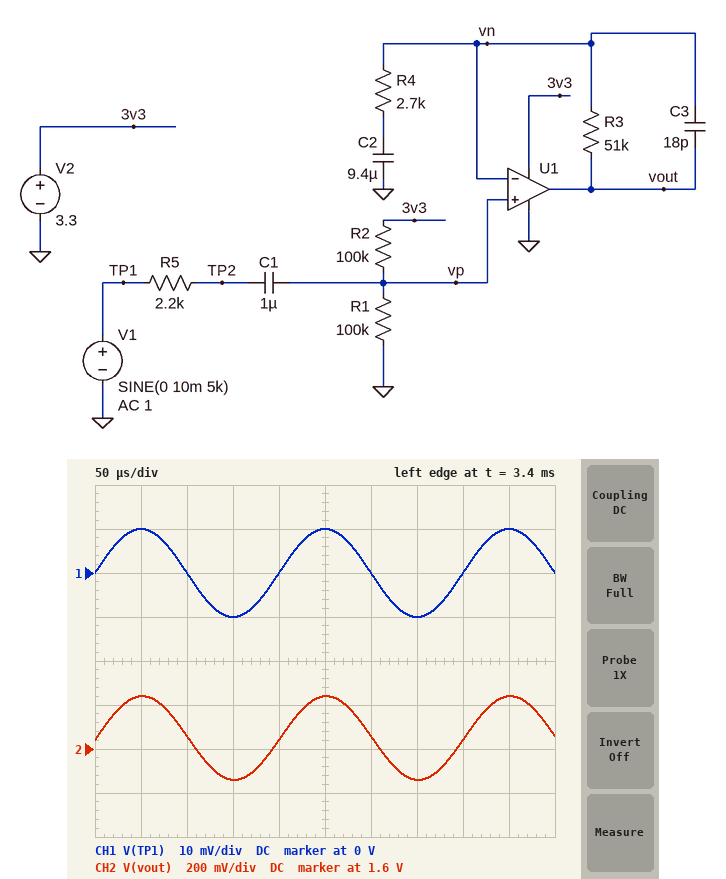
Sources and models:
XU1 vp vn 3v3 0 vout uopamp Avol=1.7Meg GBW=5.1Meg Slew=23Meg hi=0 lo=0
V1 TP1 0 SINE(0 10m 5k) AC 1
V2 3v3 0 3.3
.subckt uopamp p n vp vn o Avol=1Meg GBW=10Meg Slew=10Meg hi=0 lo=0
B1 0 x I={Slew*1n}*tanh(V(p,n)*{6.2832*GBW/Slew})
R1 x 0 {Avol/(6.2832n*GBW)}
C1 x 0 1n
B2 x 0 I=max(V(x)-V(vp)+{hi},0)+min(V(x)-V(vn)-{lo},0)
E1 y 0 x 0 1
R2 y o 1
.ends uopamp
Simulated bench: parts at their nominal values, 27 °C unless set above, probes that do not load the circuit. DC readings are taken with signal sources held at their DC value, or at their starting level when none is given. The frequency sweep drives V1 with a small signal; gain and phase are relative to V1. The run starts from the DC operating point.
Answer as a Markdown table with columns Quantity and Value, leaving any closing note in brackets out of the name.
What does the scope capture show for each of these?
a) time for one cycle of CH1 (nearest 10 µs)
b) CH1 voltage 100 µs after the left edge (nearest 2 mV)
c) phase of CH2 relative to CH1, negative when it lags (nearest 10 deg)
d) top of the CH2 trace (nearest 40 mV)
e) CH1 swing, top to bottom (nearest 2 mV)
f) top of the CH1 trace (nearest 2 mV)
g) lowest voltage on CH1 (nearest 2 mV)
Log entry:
| Quantity | Value |
|---|---|
| time for one cycle of CH1 | 200 µs |
| CH1 voltage 100 µs after the left edge | 0 V |
| phase of CH2 relative to CH1, negative when it lags | 0 deg |
| top of the CH2 trace | 1.84 V |
| CH1 swing, top to bottom | 20 mV |
| top of the CH1 trace | 10 mV |
| lowest voltage on CH1 | -10 mV |
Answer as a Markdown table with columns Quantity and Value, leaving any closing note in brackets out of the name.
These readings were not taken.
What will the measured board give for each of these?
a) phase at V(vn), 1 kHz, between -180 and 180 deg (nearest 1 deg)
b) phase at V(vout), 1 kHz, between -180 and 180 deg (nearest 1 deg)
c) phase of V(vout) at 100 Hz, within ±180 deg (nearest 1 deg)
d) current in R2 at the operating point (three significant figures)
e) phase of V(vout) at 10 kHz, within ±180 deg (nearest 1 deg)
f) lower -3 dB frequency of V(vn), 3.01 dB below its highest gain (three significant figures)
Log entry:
| Quantity | Value |
|---|---|
| phase at V(vn), 1 kHz, between -180 and 180 deg | 0 deg |
| phase at V(vout), 1 kHz, between -180 and 180 deg | 0 deg |
| phase of V(vout) at 100 Hz, within ±180 deg | 5 deg |
| current in R2 at the operating point | 16.5 µA |
| phase of V(vout) at 10 kHz, within ±180 deg | -5 deg |
| lower -3 dB frequency of V(vn), 3.01 dB below its highest gain | 3.05 Hz |
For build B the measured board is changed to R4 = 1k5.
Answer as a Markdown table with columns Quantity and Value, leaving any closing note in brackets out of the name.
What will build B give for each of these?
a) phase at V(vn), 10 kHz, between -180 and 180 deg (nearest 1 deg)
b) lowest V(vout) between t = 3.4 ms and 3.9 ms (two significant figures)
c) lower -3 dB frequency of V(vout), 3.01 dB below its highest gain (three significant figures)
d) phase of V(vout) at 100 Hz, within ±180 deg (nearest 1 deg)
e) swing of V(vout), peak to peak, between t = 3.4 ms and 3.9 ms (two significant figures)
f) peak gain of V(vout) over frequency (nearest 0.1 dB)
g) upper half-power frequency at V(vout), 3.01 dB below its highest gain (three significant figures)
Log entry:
| Quantity | Value |
|---|---|
| phase at V(vn), 10 kHz, between -180 and 180 deg | -4 deg |
| lowest V(vout) between t = 3.4 ms and 3.9 ms | 1.3 V |
| lower -3 dB frequency of V(vout), 3.01 dB below its highest gain | 12.0 Hz |
| phase of V(vout) at 100 Hz, within ±180 deg | 8 deg |
| swing of V(vout), peak to peak, between t = 3.4 ms and 3.9 ms | 670 mV |
| peak gain of V(vout) over frequency | 30.5 dB |
| upper half-power frequency at V(vout), 3.01 dB below its highest gain | 79.8 kHz |
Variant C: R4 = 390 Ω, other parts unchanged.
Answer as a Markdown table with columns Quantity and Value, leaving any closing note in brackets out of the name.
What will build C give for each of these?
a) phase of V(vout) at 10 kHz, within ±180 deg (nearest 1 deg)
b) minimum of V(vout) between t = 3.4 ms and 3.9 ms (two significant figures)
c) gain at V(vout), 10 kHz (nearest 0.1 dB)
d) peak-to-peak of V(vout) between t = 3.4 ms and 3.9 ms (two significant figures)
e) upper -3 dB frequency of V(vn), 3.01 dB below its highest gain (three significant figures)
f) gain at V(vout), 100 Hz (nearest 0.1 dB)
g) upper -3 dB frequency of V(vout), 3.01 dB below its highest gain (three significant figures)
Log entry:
| Quantity | Value |
|---|---|
| phase of V(vout) at 10 kHz, within ±180 deg | -17 deg |
| minimum of V(vout) between t = 3.4 ms and 3.9 ms | 400 mV |
| gain at V(vout), 10 kHz | 41.6 dB |
| peak-to-peak of V(vout) between t = 3.4 ms and 3.9 ms | 2.5 V |
| upper -3 dB frequency of V(vn), 3.01 dB below its highest gain | 32.8 kHz |
| gain at V(vout), 100 Hz | 41.3 dB |
| upper -3 dB frequency of V(vout), 3.01 dB below its highest gain | 31.7 kHz |
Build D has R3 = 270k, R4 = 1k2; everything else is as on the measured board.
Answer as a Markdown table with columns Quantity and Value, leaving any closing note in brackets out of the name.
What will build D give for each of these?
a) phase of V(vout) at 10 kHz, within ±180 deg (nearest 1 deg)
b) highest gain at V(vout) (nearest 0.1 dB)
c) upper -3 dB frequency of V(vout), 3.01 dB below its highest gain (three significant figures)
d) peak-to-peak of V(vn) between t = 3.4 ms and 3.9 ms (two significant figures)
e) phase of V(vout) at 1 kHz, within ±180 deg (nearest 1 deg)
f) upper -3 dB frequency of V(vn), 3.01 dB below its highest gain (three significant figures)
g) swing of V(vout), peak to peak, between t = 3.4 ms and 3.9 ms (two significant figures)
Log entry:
| Quantity | Value |
|---|---|
| phase of V(vout) at 10 kHz, within ±180 deg | -37 deg |
| highest gain at V(vout) | 46.7 dB |
| upper -3 dB frequency of V(vout), 3.01 dB below its highest gain | 13.4 kHz |
| peak-to-peak of V(vn) between t = 3.4 ms and 3.9 ms | 16 mV |
| phase of V(vout) at 1 kHz, within ±180 deg | -3 deg |
| upper -3 dB frequency of V(vn), 3.01 dB below its highest gain | 16.4 kHz |
| swing of V(vout), peak to peak, between t = 3.4 ms and 3.9 ms | 3.3 V |
